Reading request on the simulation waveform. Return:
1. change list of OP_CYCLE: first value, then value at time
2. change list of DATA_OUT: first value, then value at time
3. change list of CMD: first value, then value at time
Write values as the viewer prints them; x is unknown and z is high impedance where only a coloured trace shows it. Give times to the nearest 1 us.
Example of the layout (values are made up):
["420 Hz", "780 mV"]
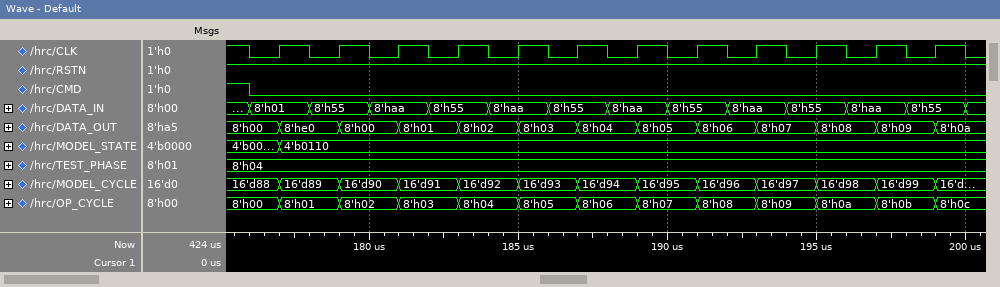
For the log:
["8'h00, 8'h01 at 177 us, 8'h02 at 179 us, 8'h03 at 181 us, 8'h04 at 183 us, 8'h05 at 185 us, 8'h06 at 187 us, 8'h07 at 189 us, 8'h08 at 191 us, 8'h09 at 193 us, 8'h0a at 195 us, 8'h0b at 197 us, 8'h0c at 199 us", "8'h00, 8'he0 at 177 us, 8'h00 at 179 us, 8'h01 at 181 us, 8'h02 at 183 us, 8'h03 at 185 us, 8'h04 at 187 us, 8'h05 at 189 us, 8'h06 at 191 us, 8'h07 at 193 us, 8'h08 at 195 us, 8'h09 at 197 us, 8'h0a at 199 us", "1, 0 at 176 us"]
